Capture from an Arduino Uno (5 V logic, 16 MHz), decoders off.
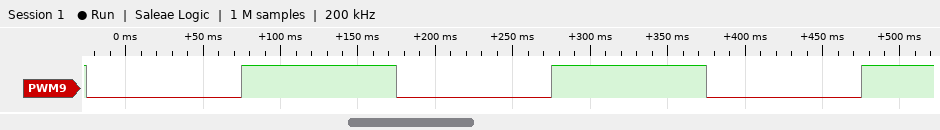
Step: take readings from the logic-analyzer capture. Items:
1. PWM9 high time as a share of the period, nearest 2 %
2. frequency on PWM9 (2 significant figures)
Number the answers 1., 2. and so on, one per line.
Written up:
1. 50 %
2. 5.0 Hz
